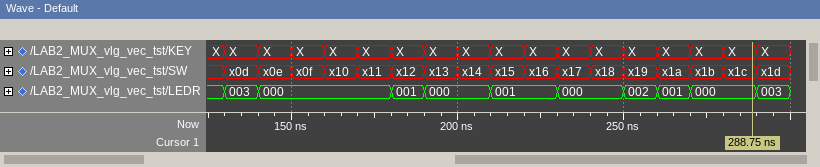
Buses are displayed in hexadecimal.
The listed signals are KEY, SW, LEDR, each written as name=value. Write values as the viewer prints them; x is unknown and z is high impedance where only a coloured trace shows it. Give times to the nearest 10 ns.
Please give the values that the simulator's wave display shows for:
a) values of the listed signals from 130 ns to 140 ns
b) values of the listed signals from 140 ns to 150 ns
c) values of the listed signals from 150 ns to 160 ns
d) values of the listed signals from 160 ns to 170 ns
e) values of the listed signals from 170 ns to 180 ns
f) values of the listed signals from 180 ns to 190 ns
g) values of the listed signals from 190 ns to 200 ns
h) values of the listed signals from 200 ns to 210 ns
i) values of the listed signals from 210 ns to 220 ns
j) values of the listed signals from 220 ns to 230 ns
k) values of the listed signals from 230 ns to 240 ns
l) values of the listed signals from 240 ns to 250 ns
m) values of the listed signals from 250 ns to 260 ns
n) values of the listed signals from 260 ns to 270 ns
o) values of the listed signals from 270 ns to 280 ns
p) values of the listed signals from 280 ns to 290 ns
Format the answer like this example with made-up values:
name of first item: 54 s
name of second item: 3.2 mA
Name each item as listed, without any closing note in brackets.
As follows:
values of the listed signals from 130 ns to 140 ns: KEY=X, SW=x0d, LEDR=003
values of the listed signals from 140 ns to 150 ns: KEY=X, SW=x0e, LEDR=000
values of the listed signals from 150 ns to 160 ns: KEY=X, SW=x0f, LEDR=000
values of the listed signals from 160 ns to 170 ns: KEY=X, SW=x10, LEDR=000
values of the listed signals from 170 ns to 180 ns: KEY=X, SW=x11, LEDR=000
values of the listed signals from 180 ns to 190 ns: KEY=X, SW=x12, LEDR=001
values of the listed signals from 190 ns to 200 ns: KEY=X, SW=x13, LEDR=000
values of the listed signals from 200 ns to 210 ns: KEY=X, SW=x14, LEDR=000
values of the listed signals from 210 ns to 220 ns: KEY=X, SW=x15, LEDR=001
values of the listed signals from 220 ns to 230 ns: KEY=X, SW=x16, LEDR=001
values of the listed signals from 230 ns to 240 ns: KEY=X, SW=x17, LEDR=000
values of the listed signals from 240 ns to 250 ns: KEY=X, SW=x18, LEDR=000
values of the listed signals from 250 ns to 260 ns: KEY=X, SW=x19, LEDR=002
values of the listed signals from 260 ns to 270 ns: KEY=X, SW=x1a, LEDR=001
values of the listed signals from 270 ns to 280 ns: KEY=X, SW=x1b, LEDR=000
values of the listed signals from 280 ns to 290 ns: KEY=X, SW=x1c, LEDR=000
